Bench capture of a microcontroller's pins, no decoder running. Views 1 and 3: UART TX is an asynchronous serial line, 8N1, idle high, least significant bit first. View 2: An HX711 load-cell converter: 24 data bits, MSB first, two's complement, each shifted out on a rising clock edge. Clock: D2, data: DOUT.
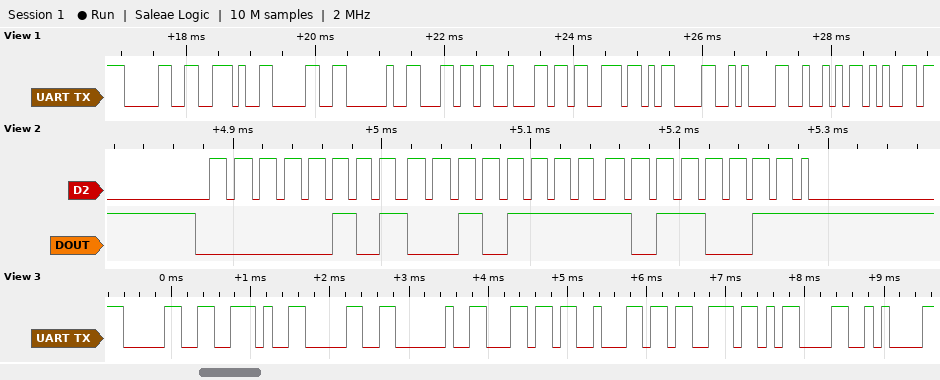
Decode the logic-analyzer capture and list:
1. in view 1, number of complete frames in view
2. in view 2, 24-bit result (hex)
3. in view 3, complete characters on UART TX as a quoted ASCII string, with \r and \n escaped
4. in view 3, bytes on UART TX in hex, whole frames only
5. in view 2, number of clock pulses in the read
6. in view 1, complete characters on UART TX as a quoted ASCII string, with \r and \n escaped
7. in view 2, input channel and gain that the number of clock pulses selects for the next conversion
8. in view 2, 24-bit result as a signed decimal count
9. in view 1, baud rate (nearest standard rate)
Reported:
11
0x052FB3
"0.0 lbs\r\n"
0x30 0x2E 0x30 0x20 0x6C 0x62 0x73 0x0D 0x0A
25
"0.0 lbs\r\nRe"
channel A, gain 128
339891
9600 baud
